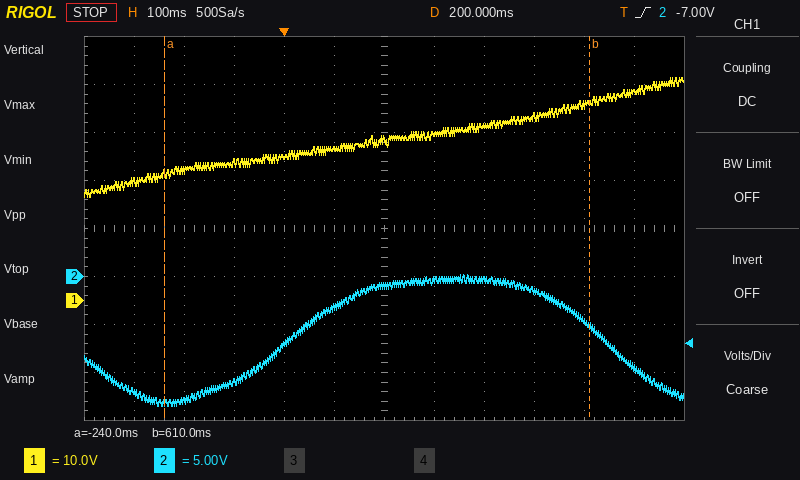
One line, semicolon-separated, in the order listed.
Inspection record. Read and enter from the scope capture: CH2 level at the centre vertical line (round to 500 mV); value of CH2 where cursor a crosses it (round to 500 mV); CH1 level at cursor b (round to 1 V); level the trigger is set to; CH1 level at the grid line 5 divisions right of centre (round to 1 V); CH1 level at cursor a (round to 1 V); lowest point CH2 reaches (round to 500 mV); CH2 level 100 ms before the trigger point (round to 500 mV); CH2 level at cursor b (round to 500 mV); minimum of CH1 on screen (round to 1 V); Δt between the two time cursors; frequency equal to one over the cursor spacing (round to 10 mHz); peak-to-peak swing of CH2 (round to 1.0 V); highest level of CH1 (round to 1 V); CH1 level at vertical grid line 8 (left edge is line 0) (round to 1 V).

-1.0 V; -13.0 V; 41 V; -7.00 V; 44 V; 26 V; -13.5 V; -11.0 V; -5.0 V; 22 V; 850 ms; 1.18 Hz; 14.0 V; 46 V; 36 V
